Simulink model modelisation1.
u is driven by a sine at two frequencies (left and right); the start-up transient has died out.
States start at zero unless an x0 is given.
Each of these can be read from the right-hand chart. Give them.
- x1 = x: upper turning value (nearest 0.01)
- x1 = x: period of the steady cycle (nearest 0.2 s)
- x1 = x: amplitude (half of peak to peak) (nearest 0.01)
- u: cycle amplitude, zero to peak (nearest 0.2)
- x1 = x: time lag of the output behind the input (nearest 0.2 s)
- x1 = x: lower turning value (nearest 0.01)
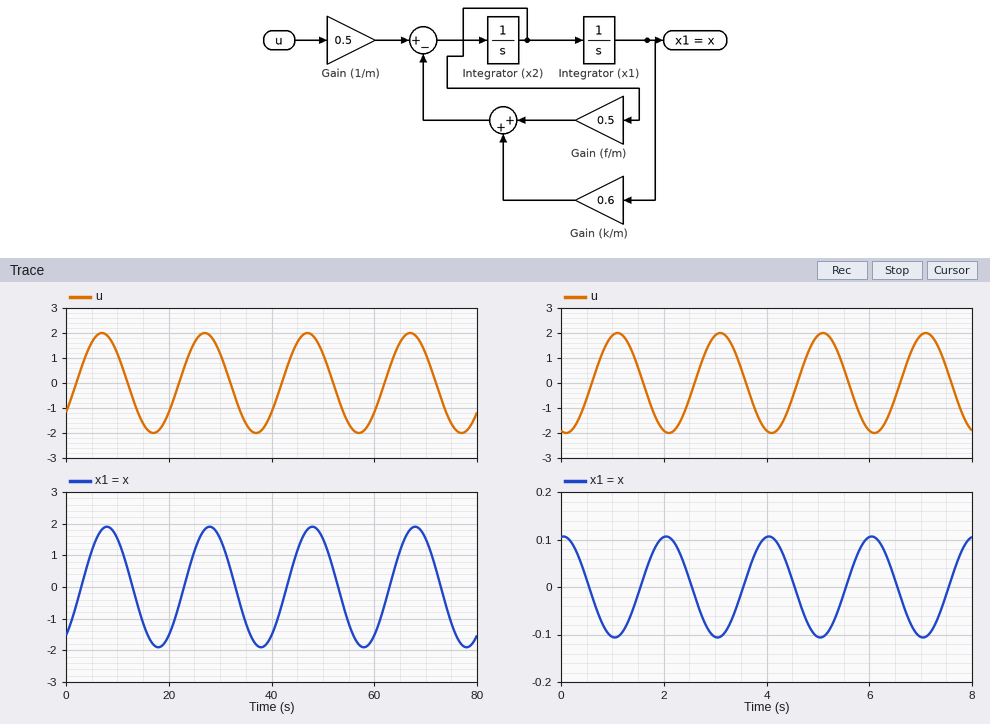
0.11
2.0 s
0.11
2.0
1.0 s
-0.11
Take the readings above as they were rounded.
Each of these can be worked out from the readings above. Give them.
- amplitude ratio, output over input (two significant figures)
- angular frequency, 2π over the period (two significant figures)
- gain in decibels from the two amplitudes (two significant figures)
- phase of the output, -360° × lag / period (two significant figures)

0.055
3.1 rad/s
-25 dB
-180°
